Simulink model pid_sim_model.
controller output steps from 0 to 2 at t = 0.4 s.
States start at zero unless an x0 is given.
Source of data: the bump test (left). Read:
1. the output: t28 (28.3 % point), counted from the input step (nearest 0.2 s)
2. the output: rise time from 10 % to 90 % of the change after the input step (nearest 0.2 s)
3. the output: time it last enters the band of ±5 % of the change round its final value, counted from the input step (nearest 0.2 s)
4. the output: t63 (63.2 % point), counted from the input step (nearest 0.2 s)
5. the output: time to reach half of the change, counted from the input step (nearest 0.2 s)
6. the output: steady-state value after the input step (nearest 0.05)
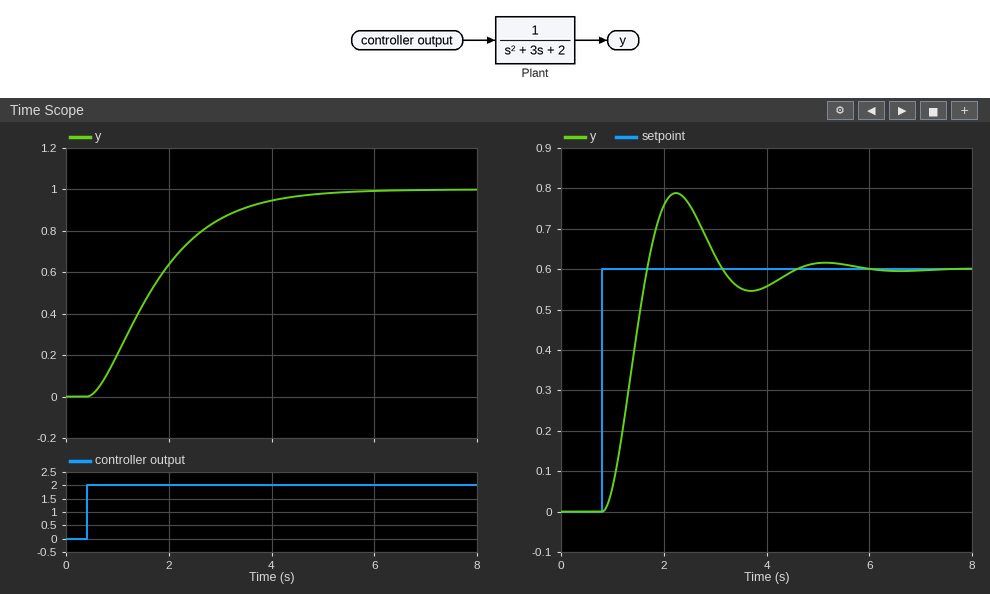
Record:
0.8 s
2.6 s
3.6 s
1.6 s
1.2 s
1.00
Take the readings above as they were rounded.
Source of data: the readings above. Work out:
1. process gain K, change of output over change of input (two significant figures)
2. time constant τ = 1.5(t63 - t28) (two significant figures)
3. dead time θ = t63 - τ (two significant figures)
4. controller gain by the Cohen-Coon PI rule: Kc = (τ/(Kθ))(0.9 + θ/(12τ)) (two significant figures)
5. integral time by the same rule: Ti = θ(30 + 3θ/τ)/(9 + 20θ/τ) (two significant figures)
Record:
0.50
1.2 s
0.40 s
5.6
0.79 s
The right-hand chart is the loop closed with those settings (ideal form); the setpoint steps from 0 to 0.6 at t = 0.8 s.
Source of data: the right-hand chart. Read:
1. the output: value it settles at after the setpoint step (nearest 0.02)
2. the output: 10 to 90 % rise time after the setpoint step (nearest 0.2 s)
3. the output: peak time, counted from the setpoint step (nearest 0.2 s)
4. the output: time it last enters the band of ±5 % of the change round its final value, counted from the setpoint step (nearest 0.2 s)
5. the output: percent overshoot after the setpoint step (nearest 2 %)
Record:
0.60
0.6 s
1.4 s
3.4 s
32 %
